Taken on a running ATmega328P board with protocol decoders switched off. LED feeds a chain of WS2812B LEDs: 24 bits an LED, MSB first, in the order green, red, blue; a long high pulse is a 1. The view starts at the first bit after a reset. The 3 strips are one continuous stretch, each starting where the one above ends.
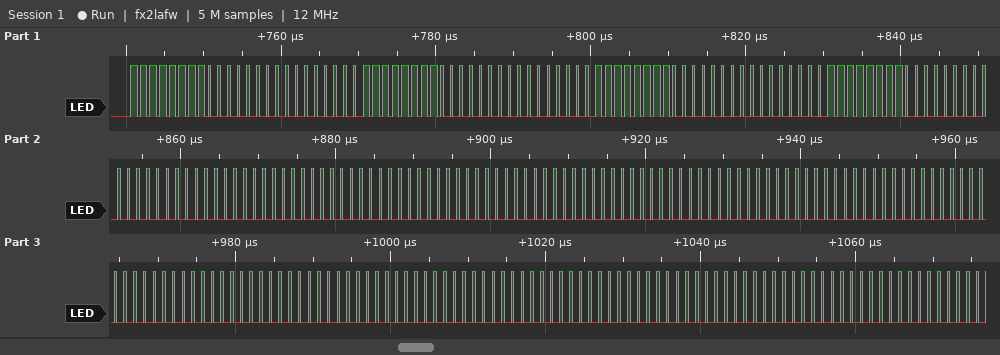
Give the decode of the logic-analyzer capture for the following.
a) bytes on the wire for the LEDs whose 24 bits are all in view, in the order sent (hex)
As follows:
FF 00 00 FF 00 00 FF 00 00 FF 00 00 00 00 00 00 00 00 00 00 00 00 00 00 00 00 00 00 00 00 00 00 00
